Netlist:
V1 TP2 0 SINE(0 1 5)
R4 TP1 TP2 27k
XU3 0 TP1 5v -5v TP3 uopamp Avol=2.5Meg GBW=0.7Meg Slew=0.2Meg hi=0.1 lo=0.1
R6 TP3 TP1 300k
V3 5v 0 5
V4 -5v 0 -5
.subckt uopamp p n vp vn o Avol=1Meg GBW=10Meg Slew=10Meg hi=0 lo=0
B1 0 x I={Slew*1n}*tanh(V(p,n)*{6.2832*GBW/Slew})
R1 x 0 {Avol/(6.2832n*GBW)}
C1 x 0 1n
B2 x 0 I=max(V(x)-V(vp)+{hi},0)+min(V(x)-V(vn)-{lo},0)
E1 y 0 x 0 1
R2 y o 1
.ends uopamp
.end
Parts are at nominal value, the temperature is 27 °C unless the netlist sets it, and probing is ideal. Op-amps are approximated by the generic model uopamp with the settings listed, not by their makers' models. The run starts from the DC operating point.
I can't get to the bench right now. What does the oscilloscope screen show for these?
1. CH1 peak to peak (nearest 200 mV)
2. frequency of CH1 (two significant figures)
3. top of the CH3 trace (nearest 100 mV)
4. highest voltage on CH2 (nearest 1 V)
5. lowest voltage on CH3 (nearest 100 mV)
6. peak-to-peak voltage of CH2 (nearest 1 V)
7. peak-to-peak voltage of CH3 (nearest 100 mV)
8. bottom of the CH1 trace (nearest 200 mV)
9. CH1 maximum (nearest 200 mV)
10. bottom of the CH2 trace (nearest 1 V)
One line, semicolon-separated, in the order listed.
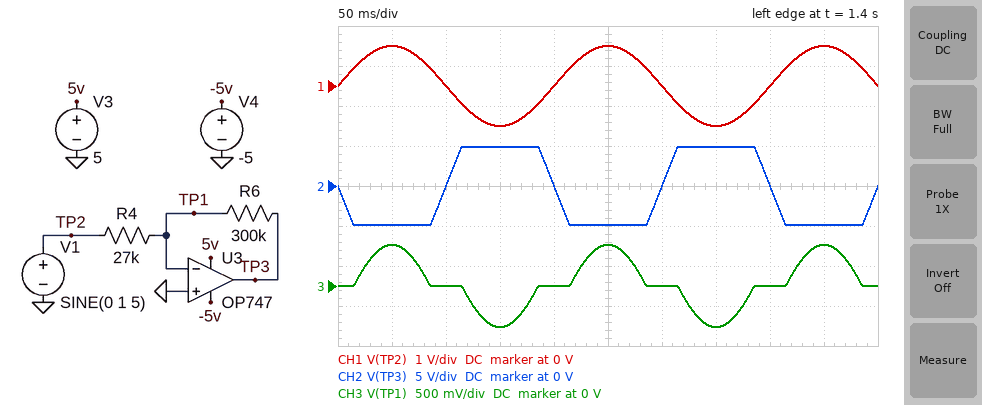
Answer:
2.0 V; 5.0 Hz; 500 mV; 5 V; -500 mV; 10 V; 1.0 V; -1.0 V; 1.0 V; -5 V
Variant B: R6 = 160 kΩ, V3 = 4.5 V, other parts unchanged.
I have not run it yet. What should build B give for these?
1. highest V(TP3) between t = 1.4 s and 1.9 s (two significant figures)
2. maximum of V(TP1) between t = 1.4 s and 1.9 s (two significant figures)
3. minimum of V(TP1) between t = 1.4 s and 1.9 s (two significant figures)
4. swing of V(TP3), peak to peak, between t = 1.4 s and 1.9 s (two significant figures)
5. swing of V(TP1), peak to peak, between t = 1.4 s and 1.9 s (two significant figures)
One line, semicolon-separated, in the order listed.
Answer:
4.4 V; 150 mV; -220 mV; 9.3 V; 370 mV
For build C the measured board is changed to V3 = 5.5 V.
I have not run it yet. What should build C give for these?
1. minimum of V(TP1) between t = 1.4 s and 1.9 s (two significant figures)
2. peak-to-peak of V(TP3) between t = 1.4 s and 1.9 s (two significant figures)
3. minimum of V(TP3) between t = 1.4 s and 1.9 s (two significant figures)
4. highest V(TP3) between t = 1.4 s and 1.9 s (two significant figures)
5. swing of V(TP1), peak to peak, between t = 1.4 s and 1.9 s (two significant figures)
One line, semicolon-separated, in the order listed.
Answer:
-470 mV; 10 V; -4.9 V; 5.4 V; 980 mV
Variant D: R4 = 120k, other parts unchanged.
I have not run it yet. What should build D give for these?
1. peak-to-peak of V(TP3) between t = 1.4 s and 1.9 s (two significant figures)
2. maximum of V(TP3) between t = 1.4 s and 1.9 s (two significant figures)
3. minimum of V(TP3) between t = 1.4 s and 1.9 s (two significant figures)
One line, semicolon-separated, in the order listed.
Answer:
5.0 V; 2.5 V; -2.5 V
